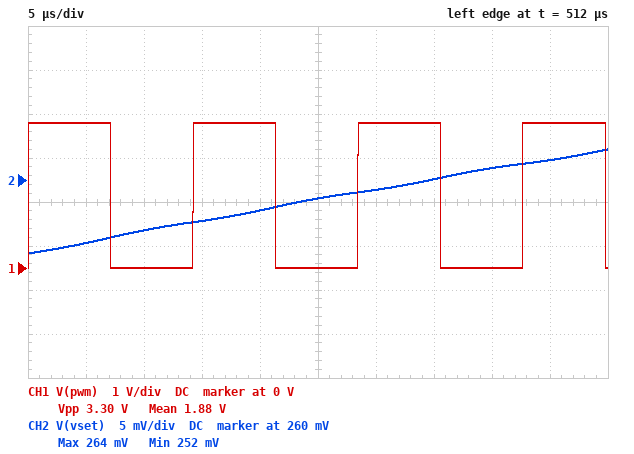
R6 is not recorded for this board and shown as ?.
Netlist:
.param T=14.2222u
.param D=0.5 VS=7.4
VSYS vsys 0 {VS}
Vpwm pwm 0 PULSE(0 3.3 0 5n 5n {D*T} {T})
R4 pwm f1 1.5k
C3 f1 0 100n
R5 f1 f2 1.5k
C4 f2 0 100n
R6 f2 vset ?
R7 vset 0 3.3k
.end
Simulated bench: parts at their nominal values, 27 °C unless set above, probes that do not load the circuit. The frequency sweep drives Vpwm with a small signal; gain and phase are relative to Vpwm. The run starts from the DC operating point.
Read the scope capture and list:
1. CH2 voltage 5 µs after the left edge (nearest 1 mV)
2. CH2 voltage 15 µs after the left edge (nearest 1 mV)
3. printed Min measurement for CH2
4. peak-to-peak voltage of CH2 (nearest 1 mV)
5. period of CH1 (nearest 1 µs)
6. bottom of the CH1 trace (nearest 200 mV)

253 mV
255 mV
252 mV
12 mV
14 µs
0 V
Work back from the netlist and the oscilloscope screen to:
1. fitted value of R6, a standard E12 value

10 kΩ
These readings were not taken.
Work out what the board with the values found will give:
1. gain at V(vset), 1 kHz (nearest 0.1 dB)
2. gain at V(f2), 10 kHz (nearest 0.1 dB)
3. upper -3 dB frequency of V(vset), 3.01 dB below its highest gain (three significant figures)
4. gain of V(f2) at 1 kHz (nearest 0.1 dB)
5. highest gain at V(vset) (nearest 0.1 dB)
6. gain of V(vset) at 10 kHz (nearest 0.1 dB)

-21.5 dB
-39.3 dB
477 Hz
-9.4 dB
-13.9 dB
-51.4 dB
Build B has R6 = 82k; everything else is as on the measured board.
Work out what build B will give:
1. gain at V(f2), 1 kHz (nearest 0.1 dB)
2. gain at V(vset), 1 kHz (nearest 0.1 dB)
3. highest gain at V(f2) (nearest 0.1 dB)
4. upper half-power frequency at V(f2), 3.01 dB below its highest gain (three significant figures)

-9.1 dB
-37.3 dB
-0.3 dB
410 Hz
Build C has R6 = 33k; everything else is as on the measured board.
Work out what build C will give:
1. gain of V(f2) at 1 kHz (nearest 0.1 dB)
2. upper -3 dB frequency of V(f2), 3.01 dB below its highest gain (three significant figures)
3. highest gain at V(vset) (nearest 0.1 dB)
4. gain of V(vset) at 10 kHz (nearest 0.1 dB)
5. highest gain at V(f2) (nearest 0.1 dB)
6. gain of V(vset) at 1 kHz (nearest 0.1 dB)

-9.2 dB
427 Hz
-21.5 dB
-60.1 dB
-0.7 dB
-30.0 dB
